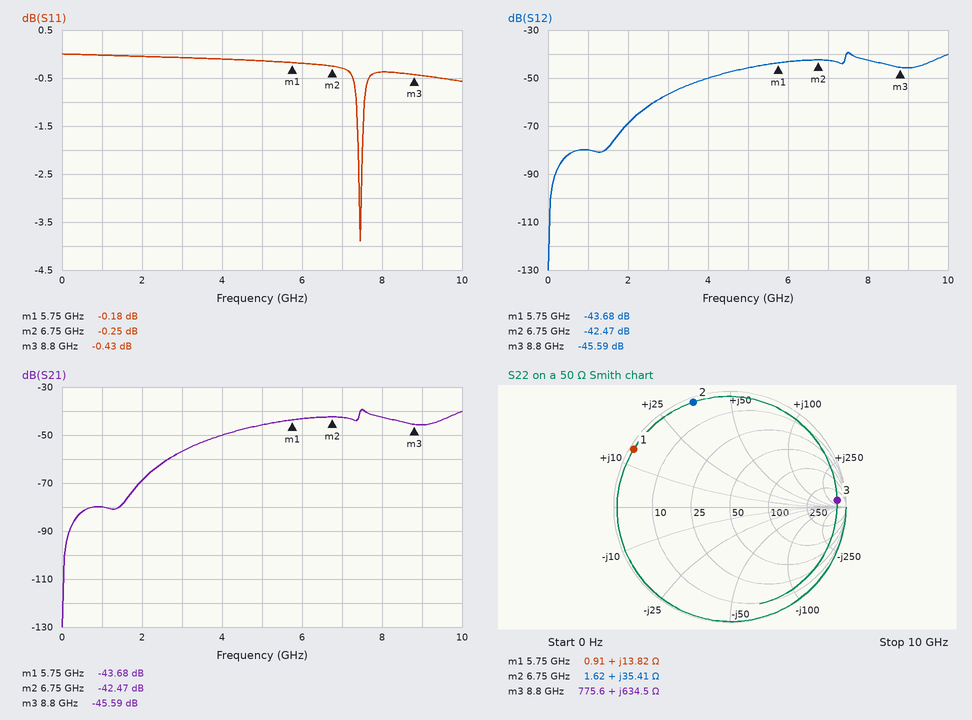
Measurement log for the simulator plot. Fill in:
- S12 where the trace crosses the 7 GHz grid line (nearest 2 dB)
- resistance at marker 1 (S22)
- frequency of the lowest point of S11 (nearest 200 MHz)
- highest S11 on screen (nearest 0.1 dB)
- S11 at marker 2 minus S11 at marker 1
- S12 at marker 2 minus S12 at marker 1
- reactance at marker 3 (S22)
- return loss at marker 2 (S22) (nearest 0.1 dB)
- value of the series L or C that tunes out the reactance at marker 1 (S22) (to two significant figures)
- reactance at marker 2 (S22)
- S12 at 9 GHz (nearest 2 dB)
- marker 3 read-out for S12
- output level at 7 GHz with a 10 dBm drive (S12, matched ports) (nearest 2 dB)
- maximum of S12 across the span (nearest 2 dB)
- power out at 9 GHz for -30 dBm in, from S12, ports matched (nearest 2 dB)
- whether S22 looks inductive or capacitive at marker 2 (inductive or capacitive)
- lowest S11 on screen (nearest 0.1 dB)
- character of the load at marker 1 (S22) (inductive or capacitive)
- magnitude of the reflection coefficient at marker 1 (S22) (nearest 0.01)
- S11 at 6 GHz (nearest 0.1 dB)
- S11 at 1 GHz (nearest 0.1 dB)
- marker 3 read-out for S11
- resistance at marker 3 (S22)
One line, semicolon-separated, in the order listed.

-42 dB; 0.91 Ω; 7.4 GHz; 0.0 dB; -0.07 dB; 1.21 dB; +634.5 Ω; 0.4 dB; 2.0 pF; +35.41 Ω; -46 dB; -45.59 dB; -32 dBm; -40 dB; -76 dBm; inductive; -3.9 dB; inductive; 0.97; -0.2 dB; 0.0 dB; -0.43 dB; 775.6 Ω
